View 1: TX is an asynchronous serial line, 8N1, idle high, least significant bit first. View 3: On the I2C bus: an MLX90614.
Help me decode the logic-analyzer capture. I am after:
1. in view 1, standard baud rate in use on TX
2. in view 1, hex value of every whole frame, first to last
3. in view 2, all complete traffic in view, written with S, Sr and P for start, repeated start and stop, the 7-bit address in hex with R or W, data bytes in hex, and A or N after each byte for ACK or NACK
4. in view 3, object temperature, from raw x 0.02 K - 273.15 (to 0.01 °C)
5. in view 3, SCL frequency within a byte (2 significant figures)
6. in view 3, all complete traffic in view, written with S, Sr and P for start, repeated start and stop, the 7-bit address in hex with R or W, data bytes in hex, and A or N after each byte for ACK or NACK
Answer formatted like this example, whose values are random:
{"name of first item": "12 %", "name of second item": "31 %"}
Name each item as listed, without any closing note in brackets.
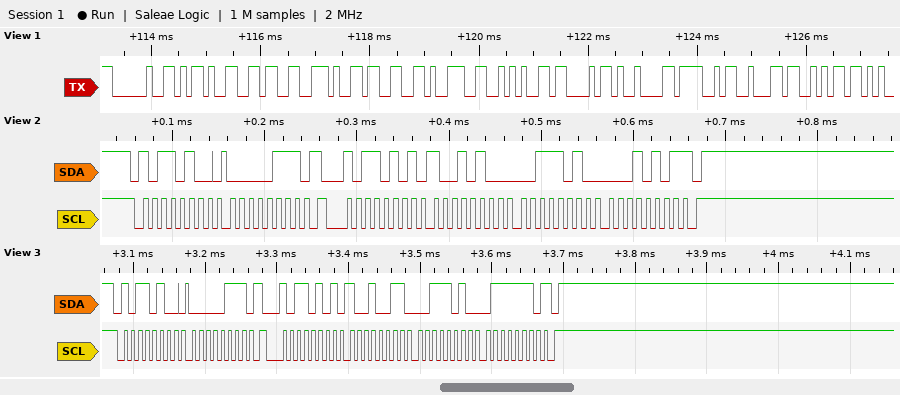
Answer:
{"in view 1, standard baud rate in use on TX": "9600 baud", "in view 1, hex value of every whole frame, first to last": "20 2D 36 2E 33 39 2A 43 09 4F 62 6A", "in view 2, all complete traffic in view, written with S, Sr and P for start, repeated start and stop, the 7-bit address in hex with R or W, data bytes in hex, and A or N after each byte for ACK or NACK": "S 5AW A 07 A Sr 5AR A 94 A 3A A 15 N P", "in view 3, object temperature, from raw x 0.02 K - 273.15": "26.75 °C", "in view 3, SCL frequency within a byte": "100 kHz", "in view 3, all complete traffic in view, written with S, Sr and P for start, repeated start and stop, the 7-bit address in hex with R or W, data bytes in hex, and A or N after each byte for ACK or NACK": "S 5AW A 07 A Sr 5AR A 93 A 3A A 7E N P"}
